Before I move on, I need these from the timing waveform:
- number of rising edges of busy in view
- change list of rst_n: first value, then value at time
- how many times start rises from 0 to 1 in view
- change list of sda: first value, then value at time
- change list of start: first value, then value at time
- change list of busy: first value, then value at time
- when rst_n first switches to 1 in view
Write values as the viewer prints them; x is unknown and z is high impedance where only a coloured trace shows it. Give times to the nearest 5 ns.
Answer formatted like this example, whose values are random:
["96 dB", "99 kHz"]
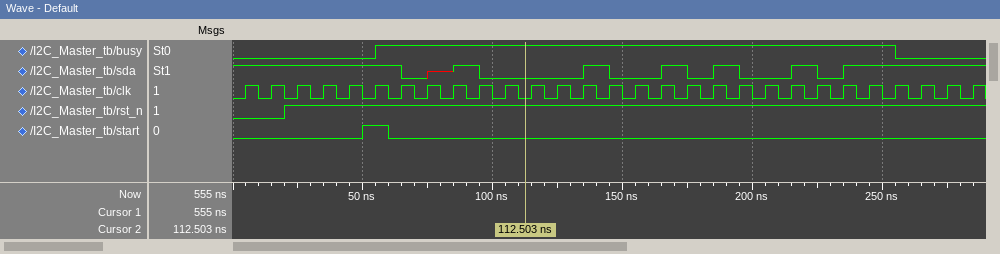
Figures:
["1", "0, 1 at 20 ns", "1", "1, 0 at 65 ns, x at 75 ns, 1 at 85 ns, 0 at 95 ns, 1 at 135 ns, 0 at 145 ns, 1 at 165 ns, 0 at 175 ns, 1 at 185 ns, 0 at 195 ns, 1 at 215 ns, 0 at 225 ns, 1 at 235 ns", "0, 1 at 50 ns, 0 at 60 ns", "0, 1 at 55 ns, 0 at 255 ns", "20 ns"]
